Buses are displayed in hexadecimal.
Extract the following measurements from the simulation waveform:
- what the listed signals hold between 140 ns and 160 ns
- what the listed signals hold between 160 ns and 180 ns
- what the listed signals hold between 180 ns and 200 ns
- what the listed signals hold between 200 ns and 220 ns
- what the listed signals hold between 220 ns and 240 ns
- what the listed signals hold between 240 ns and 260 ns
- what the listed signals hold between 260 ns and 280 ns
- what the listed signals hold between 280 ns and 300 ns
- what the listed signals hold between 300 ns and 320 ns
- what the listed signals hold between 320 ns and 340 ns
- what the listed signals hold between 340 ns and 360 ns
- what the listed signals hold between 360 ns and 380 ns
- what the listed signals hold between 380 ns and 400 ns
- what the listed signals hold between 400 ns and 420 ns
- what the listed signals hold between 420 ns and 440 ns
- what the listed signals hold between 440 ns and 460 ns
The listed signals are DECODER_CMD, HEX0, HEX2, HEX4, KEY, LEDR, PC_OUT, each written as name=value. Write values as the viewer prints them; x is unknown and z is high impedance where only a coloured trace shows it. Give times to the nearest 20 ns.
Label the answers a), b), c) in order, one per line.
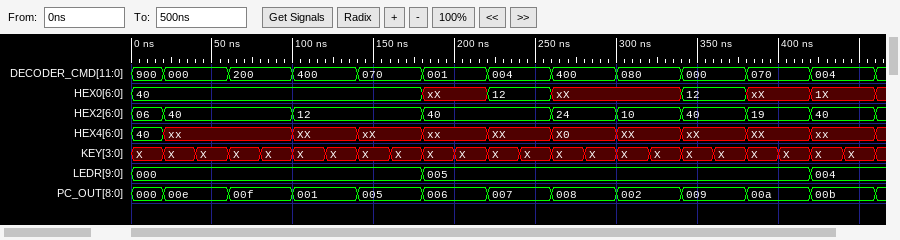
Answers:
a) DECODER_CMD=070, HEX0=40, HEX2=12, HEX4=xX, KEY=X, LEDR=000, PC_OUT=005
b) DECODER_CMD=070, HEX0=40, HEX2=12, HEX4=xX, KEY=X, LEDR=000, PC_OUT=005
c) DECODER_CMD=001, HEX0=xX, HEX2=40, HEX4=xx, KEY=X, LEDR=005, PC_OUT=006
d) DECODER_CMD=001, HEX0=xX, HEX2=40, HEX4=xx, KEY=X, LEDR=005, PC_OUT=006
e) DECODER_CMD=004, HEX0=12, HEX2=40, HEX4=XX, KEY=X, LEDR=005, PC_OUT=007
f) DECODER_CMD=004, HEX0=12, HEX2=40, HEX4=XX, KEY=X, LEDR=005, PC_OUT=007
g) DECODER_CMD=400, HEX0=xX, HEX2=24, HEX4=X0, KEY=X, LEDR=005, PC_OUT=008
h) DECODER_CMD=400, HEX0=xX, HEX2=24, HEX4=X0, KEY=X, LEDR=005, PC_OUT=008
i) DECODER_CMD=080, HEX0=xX, HEX2=10, HEX4=XX, KEY=X, LEDR=005, PC_OUT=002
j) DECODER_CMD=080, HEX0=xX, HEX2=10, HEX4=XX, KEY=X, LEDR=005, PC_OUT=002
k) DECODER_CMD=000, HEX0=12, HEX2=40, HEX4=xX, KEY=X, LEDR=005, PC_OUT=009
l) DECODER_CMD=000, HEX0=12, HEX2=40, HEX4=xX, KEY=X, LEDR=005, PC_OUT=009
m) DECODER_CMD=070, HEX0=xX, HEX2=19, HEX4=XX, KEY=X, LEDR=005, PC_OUT=00a
n) DECODER_CMD=070, HEX0=xX, HEX2=19, HEX4=XX, KEY=X, LEDR=005, PC_OUT=00a
o) DECODER_CMD=004, HEX0=1X, HEX2=40, HEX4=xx, KEY=X, LEDR=004, PC_OUT=00b
p) DECODER_CMD=004, HEX0=1X, HEX2=40, HEX4=xx, KEY=X, LEDR=004, PC_OUT=00b
